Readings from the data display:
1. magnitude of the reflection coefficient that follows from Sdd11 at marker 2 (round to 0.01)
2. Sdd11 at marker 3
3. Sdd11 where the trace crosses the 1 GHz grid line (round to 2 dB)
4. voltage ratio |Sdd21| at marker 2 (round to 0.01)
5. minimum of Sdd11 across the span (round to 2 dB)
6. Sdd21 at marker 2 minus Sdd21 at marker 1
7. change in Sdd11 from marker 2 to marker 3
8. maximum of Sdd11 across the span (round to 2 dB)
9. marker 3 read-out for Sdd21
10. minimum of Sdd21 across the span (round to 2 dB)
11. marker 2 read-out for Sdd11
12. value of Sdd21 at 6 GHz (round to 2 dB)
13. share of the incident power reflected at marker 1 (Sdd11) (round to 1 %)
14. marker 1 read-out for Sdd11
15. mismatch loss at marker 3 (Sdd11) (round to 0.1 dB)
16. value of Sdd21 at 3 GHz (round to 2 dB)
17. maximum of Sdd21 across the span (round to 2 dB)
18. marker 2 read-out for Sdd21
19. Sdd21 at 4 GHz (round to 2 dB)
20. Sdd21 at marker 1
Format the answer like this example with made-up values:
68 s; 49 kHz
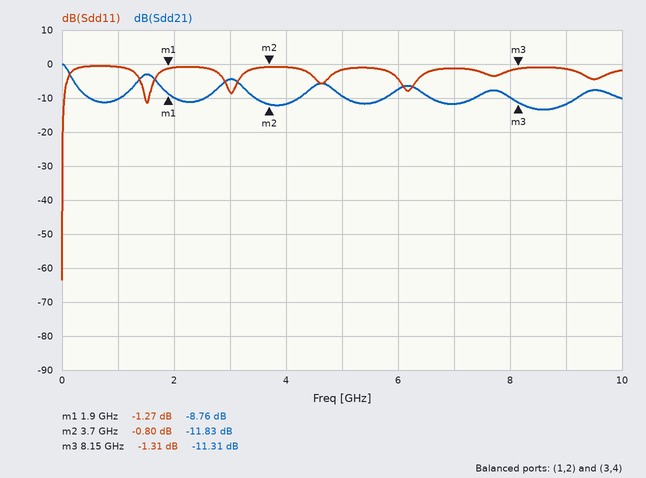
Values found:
0.91; -1.31 dB; 0 dB; 0.26; -64 dB; -3.07 dB; -0.51 dB; 0 dB; -11.31 dB; -14 dB; -0.80 dB; -8 dB; 75 %; -1.27 dB; 5.8 dB; -4 dB; 0 dB; -11.83 dB; -12 dB; -8.76 dB
